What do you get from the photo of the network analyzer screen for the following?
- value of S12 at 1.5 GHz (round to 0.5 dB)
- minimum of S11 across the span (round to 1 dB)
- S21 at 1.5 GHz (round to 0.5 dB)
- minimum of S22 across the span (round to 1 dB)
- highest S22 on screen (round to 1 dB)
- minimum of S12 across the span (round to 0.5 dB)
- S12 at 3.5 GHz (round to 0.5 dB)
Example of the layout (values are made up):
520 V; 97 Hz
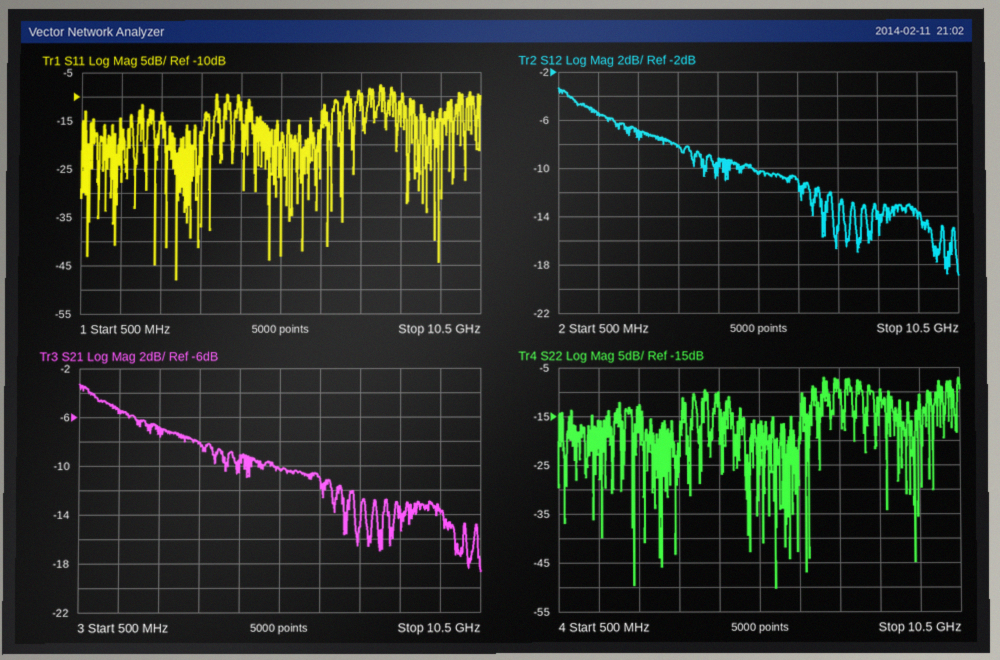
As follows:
-5.5 dB; -48 dB; -5.5 dB; -50 dB; -7 dB; -19.0 dB; -8.0 dB
